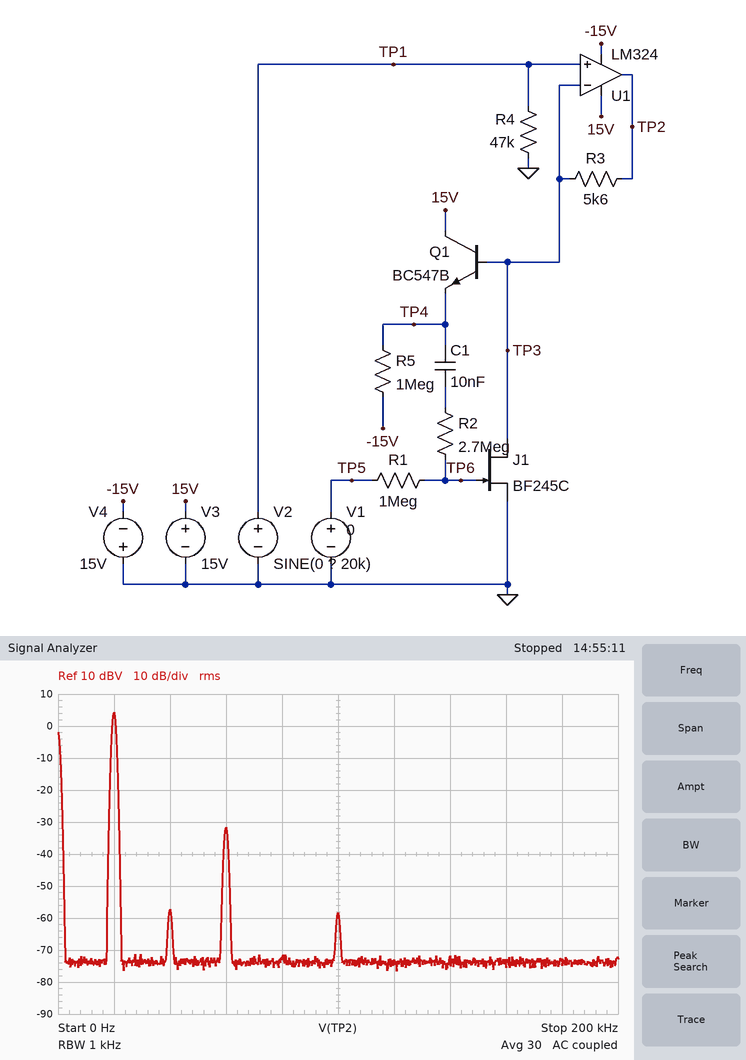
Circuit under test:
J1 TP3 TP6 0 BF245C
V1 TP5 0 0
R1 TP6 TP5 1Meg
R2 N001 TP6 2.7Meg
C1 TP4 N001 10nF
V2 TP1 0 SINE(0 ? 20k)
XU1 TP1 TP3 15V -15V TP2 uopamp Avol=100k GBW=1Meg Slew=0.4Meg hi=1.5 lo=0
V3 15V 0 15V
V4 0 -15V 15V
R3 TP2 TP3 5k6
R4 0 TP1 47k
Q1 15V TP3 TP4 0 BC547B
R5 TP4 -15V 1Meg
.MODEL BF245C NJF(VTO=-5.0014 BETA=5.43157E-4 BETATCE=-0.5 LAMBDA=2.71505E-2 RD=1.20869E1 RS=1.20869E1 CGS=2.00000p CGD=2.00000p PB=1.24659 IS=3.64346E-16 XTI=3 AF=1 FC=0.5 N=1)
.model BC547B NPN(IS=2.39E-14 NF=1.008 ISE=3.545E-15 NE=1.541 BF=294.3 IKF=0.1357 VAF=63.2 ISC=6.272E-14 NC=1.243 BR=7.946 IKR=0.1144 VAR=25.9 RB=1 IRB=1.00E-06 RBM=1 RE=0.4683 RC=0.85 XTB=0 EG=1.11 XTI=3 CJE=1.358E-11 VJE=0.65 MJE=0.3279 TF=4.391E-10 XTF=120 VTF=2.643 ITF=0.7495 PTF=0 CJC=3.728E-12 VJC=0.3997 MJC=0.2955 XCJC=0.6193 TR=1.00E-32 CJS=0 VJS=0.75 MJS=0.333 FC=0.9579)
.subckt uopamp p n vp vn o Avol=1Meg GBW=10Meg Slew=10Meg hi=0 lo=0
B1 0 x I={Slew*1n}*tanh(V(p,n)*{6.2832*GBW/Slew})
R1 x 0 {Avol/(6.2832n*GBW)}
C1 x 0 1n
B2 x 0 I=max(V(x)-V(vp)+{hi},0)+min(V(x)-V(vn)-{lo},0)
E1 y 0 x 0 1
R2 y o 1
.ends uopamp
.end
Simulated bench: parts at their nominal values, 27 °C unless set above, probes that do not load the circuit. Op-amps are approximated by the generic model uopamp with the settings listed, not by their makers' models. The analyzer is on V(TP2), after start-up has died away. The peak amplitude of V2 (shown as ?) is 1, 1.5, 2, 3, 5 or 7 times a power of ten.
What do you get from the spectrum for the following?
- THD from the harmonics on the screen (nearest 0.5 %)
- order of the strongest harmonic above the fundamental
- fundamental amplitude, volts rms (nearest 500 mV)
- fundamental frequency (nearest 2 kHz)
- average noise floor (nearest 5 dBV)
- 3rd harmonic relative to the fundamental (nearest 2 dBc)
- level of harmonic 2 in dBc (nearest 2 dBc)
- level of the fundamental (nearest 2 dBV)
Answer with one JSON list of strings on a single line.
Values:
["1.5 %", "3", "1.5 V", "20 kHz", "-75 dBV", "-36 dBc", "-62 dBc", "4 dBV"]
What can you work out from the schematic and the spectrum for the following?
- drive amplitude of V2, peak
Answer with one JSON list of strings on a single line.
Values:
["100 mV"]
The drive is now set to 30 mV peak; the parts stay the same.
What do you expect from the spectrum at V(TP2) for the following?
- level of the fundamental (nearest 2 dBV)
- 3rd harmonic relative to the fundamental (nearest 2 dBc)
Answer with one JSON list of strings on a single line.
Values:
["-6 dBV", "-58 dBc"]
